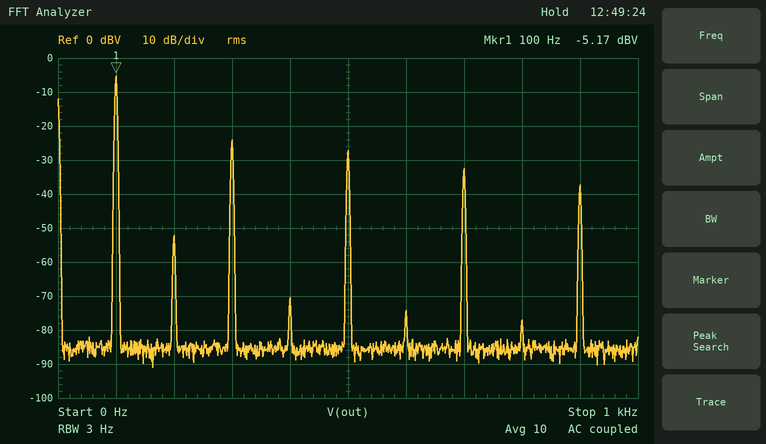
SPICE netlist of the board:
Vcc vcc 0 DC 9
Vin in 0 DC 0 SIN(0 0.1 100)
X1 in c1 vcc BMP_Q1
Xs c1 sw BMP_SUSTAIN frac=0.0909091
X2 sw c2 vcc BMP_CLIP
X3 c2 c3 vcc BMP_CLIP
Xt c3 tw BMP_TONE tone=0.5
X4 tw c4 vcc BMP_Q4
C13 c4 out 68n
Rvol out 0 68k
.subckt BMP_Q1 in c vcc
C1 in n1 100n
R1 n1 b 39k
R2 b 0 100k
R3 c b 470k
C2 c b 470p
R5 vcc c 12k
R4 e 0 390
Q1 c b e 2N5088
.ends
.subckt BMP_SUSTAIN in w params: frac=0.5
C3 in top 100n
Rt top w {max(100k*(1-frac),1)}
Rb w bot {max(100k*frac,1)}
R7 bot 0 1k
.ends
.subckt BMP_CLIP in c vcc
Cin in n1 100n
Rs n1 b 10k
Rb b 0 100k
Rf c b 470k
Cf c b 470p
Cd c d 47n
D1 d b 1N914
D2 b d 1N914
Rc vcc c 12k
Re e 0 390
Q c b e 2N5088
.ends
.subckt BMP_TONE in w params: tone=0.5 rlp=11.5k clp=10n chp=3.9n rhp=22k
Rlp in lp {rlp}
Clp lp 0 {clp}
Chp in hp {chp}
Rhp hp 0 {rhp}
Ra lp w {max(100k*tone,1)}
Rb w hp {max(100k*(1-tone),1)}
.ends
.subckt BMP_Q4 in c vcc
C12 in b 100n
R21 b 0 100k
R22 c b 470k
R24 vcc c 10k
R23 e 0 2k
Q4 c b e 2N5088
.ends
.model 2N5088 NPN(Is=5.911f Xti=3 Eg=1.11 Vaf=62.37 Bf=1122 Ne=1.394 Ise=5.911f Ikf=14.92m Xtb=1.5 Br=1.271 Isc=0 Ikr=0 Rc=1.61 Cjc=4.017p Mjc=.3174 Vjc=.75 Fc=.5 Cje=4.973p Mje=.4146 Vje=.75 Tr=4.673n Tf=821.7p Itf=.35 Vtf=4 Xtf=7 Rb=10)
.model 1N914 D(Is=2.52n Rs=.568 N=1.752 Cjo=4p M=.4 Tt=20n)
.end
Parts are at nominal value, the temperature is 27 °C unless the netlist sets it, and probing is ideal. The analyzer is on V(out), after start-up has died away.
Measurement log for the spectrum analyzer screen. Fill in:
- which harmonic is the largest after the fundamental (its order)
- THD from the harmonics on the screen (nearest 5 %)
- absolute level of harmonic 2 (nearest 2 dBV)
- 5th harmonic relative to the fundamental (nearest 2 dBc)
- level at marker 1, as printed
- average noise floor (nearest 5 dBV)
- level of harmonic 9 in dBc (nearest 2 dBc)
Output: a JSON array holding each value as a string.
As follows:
["3", "15 %", "-52 dBV", "-22 dBc", "-5.17 dBV", "-85 dBV", "-32 dBc"]
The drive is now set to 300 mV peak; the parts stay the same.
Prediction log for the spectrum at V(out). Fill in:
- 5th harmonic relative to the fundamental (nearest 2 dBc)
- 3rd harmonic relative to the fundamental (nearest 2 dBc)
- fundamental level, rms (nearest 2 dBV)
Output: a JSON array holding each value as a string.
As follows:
["-24 dBc", "-16 dBc", "-2 dBV"]
